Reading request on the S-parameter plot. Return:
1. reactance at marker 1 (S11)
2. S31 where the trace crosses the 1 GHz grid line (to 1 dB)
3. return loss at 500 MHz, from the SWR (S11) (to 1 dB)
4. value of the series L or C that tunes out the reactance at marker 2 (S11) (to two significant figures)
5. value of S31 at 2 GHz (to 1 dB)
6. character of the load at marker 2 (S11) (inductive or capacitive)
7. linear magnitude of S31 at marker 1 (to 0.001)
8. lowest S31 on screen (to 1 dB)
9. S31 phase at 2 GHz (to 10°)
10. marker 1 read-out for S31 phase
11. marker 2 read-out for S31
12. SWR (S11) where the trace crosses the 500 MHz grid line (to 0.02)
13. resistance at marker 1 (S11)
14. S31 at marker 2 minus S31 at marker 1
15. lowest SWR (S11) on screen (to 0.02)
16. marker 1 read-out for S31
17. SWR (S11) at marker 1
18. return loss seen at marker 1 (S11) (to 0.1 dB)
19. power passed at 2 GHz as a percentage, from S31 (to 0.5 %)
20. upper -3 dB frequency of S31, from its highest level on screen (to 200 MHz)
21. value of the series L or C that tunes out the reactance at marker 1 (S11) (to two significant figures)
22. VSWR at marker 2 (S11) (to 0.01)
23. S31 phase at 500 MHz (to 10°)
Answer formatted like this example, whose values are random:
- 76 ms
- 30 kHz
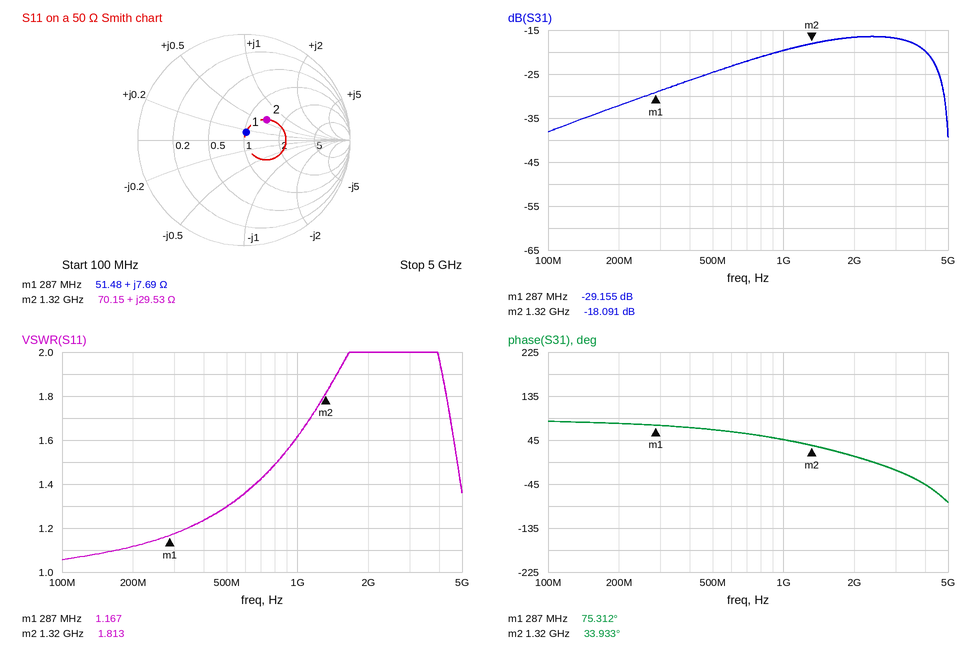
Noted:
- +7.69 Ω
- -20 dB
- 18 dB
- 4.1 pF
- -17 dB
- inductive
- 0.035
- -39 dB
- 10°
- 75.312°
- -18.091 dB
- 1.30
- 51.48 Ω
- 11.064 dB
- 1.06
- -29.155 dB
- 1.167
- 22.3 dB
- 2.0 %
- 4.0 GHz
- 72 pF
- 1.81
- 70°
